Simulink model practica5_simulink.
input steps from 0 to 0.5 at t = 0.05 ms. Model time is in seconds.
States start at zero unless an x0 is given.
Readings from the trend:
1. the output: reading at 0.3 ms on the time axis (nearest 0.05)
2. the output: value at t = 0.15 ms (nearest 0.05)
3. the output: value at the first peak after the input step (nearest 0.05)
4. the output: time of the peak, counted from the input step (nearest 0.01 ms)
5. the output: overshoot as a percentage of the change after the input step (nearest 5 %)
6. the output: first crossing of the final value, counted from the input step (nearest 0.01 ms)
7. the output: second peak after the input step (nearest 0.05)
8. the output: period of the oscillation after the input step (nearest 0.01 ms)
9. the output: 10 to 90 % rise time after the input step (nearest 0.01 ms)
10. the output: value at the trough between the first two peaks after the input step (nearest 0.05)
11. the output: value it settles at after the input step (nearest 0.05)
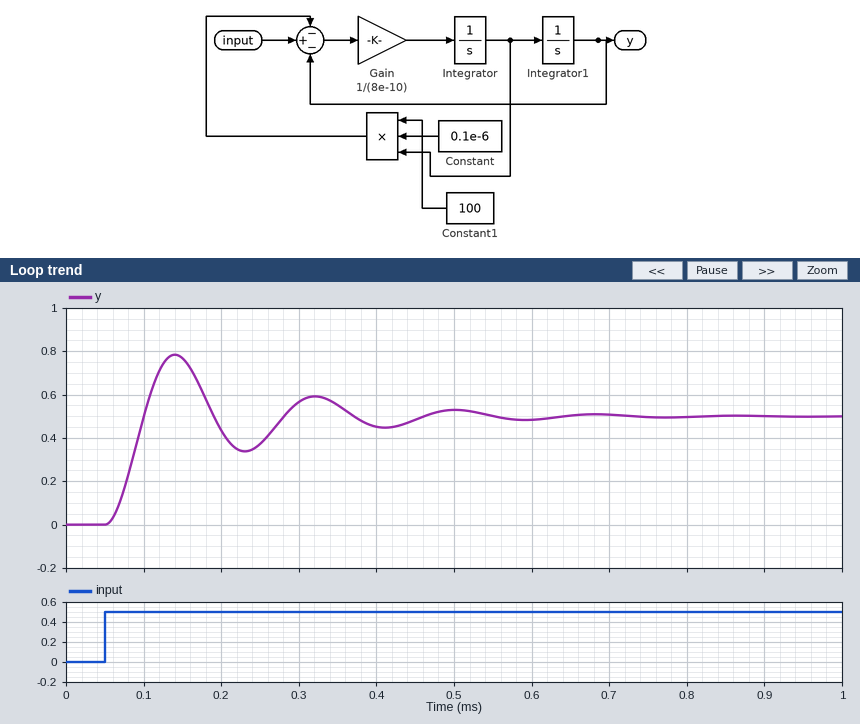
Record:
0.55
0.75
0.80
0.09 ms
55 %
0.05 ms
0.60
0.18 ms
0.03 ms
0.35
0.50
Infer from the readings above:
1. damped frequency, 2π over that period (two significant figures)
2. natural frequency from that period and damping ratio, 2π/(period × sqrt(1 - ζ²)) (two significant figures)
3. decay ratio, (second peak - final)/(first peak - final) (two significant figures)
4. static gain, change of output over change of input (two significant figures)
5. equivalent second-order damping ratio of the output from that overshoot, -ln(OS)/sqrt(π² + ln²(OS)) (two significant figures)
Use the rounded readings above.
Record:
35 rad/ms
36 rad/ms
0.33
1.0
0.19
